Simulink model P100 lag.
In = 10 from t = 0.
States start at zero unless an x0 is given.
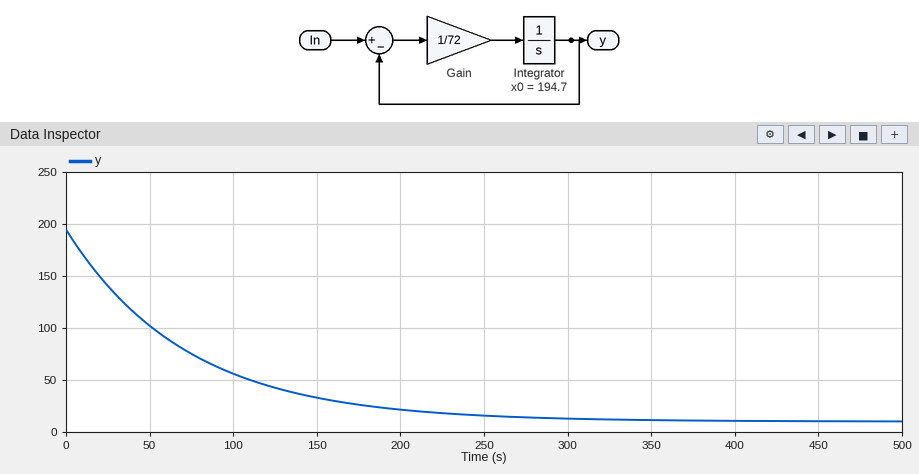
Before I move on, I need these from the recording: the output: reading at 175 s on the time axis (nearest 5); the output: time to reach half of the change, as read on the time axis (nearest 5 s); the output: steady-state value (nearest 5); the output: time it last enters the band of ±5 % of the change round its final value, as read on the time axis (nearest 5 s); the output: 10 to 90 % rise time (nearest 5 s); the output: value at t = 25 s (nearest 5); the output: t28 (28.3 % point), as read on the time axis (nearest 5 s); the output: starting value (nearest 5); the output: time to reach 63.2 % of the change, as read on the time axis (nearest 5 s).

25
50 s
10
215 s
160 s
140
25 s
195
70 s
